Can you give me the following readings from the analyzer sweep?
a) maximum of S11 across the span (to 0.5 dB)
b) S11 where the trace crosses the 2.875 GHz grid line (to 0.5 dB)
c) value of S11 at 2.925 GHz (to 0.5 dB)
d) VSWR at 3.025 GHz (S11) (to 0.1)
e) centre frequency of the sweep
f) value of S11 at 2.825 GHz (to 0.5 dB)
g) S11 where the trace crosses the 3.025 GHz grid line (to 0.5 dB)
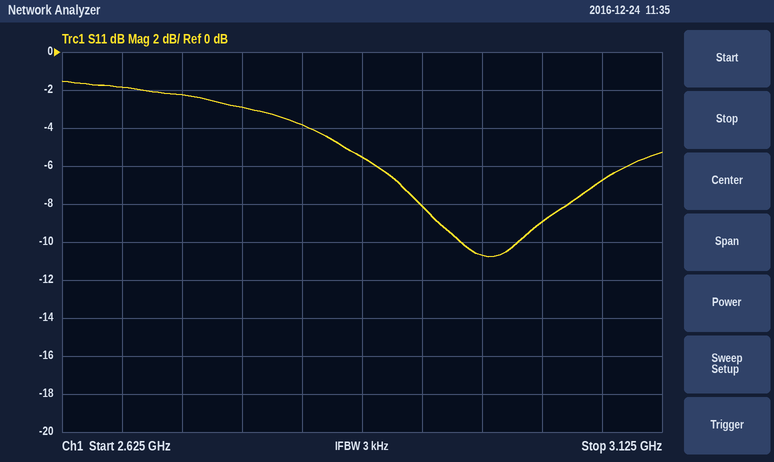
-1.5 dB
-5.5 dB
-8.0 dB
2.1
2.875 GHz
-4.0 dB
-9.0 dB
